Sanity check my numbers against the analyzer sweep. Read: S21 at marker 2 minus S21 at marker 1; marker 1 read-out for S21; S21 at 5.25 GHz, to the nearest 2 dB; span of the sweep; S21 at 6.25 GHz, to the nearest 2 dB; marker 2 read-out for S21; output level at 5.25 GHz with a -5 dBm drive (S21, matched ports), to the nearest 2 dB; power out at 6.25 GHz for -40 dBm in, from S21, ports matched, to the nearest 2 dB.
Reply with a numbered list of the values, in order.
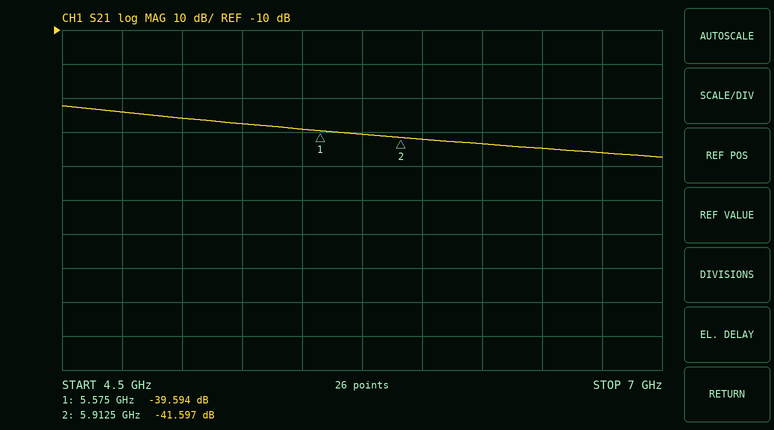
1. -2.003 dB
2. -39.594 dB
3. -38 dB
4. 2.5 GHz
5. -44 dB
6. -41.597 dB
7. -42 dBm
8. -84 dBm
